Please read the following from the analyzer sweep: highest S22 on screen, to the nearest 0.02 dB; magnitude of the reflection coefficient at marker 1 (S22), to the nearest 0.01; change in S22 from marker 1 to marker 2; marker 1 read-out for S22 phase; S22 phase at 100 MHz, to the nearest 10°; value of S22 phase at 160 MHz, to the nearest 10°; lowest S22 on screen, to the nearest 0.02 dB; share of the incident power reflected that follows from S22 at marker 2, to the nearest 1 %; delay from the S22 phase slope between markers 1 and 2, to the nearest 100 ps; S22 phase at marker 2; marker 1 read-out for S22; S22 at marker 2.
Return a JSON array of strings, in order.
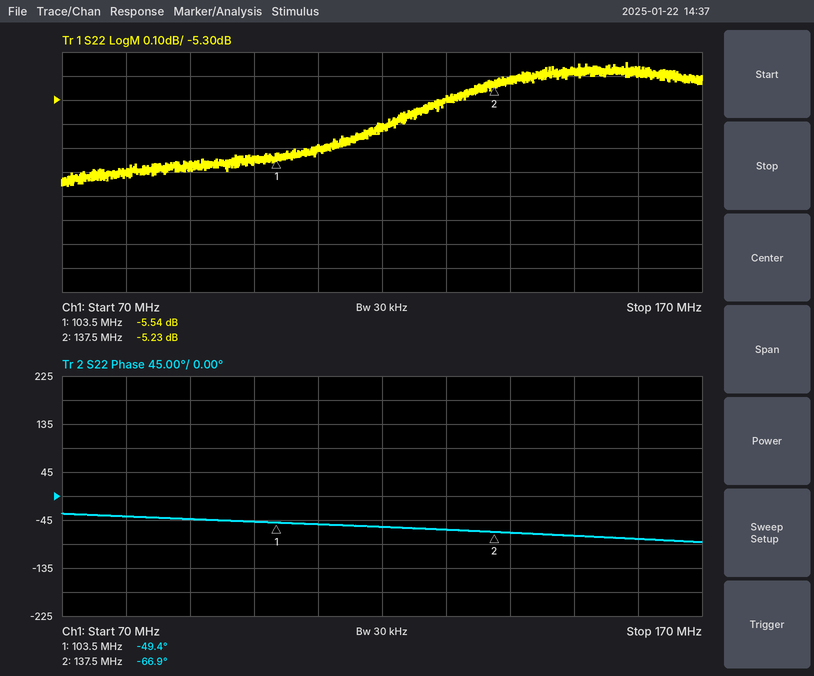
["-5.14 dB", "0.53", "0.31 dB", "-49.4°", "-50°", "-80°", "-5.66 dB", "30 %", "1.4 ns", "-66.9°", "-5.54 dB", "-5.23 dB"]
